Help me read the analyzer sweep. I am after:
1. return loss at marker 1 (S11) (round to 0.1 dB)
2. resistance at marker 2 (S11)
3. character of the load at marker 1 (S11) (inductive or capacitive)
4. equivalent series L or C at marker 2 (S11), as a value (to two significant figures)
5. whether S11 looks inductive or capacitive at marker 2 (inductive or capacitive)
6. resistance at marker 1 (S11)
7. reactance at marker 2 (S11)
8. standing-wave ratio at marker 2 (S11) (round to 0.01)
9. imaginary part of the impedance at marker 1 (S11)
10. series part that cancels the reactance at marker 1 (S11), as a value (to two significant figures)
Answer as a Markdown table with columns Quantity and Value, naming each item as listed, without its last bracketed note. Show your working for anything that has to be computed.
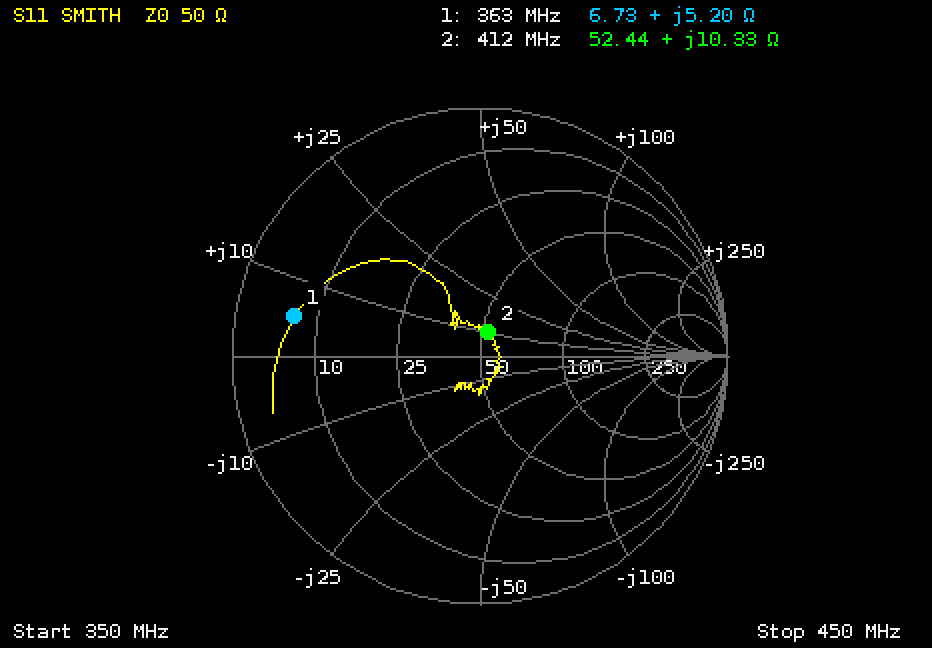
| Quantity | Value |
|---|---|
| return loss at marker 1 (S11) | 2.3 dB |
| resistance at marker 2 | 52.44 Ω |
| character of the load at marker 1 (S11) | inductive |
| equivalent series L or C at marker 2 (S11), as a value | L = 10.33 Ω/(2π × 412 MHz) ≈ 4.0 nH |
| whether S11 looks inductive or capacitive at marker 2 | inductive |
| resistance at marker 1 | 6.73 Ω |
| reactance at marker 2 | +10.33 Ω |
| standing-wave ratio at marker 2 (S11) | 1.23 |
| imaginary part of the impedance at marker 1 | +5.20 Ω |
| series part that cancels the reactance at marker 1 (S11), as a value | C = 1/(2π × 363 MHz × 5.2 Ω) ≈ 84 pF |
